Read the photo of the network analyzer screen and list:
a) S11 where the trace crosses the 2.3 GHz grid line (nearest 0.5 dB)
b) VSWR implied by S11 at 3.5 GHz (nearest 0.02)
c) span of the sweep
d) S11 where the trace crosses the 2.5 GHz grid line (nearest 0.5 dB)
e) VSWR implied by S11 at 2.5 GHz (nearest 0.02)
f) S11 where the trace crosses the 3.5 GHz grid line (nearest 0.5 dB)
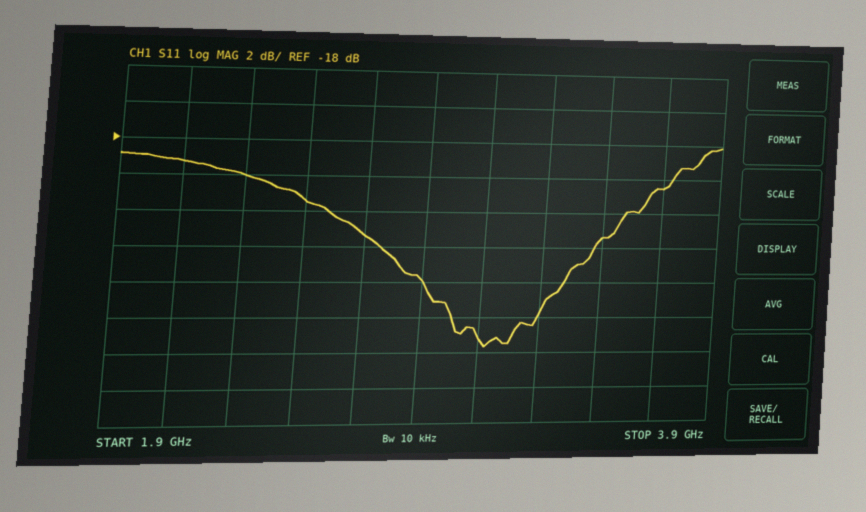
-20.0 dB
1.14
2 GHz
-21.5 dB
1.18
-23.5 dB
